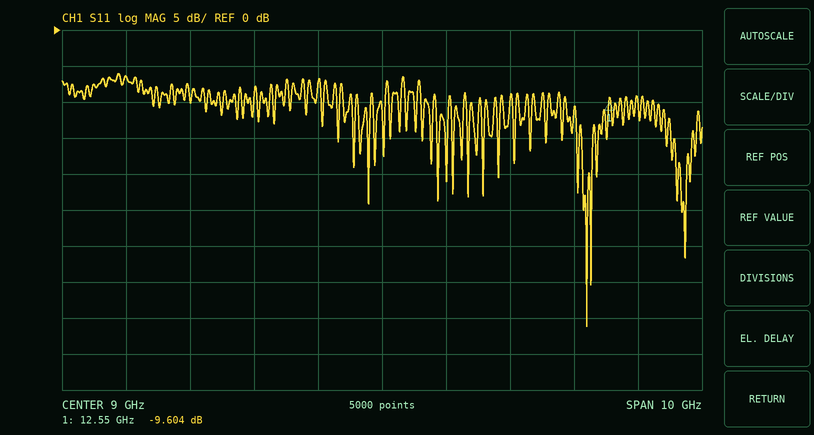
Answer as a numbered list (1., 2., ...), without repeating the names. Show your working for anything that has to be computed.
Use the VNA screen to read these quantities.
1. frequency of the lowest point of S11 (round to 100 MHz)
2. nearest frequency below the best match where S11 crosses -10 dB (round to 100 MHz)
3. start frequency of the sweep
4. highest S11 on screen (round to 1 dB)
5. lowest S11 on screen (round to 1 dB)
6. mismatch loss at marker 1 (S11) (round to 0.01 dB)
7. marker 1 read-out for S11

1. 12.2 GHz
2. 11.9 GHz
3. 4 GHz
4. -6 dB
5. -41 dB
6. −10 log10(1 − 10^(-9.604/10)) ≈ 0.50 dB
7. -9.604 dB
